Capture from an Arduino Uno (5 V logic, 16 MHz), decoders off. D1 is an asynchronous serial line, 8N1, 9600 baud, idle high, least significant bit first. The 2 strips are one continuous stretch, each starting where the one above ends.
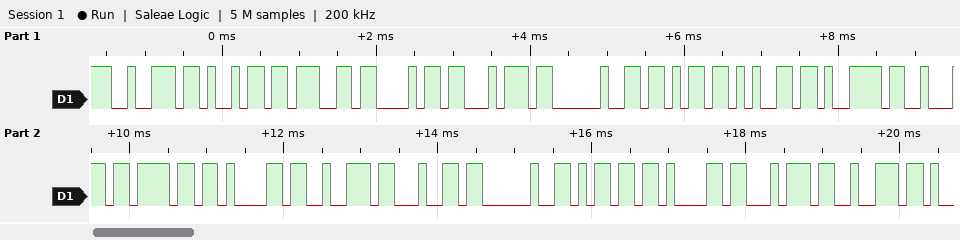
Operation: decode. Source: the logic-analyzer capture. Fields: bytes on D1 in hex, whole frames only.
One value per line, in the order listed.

72 69 67 68 74 20 6B 65 79 62 6F 61 72 64 20 6D 61 74 72
